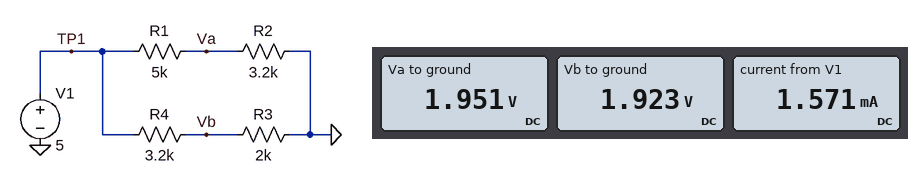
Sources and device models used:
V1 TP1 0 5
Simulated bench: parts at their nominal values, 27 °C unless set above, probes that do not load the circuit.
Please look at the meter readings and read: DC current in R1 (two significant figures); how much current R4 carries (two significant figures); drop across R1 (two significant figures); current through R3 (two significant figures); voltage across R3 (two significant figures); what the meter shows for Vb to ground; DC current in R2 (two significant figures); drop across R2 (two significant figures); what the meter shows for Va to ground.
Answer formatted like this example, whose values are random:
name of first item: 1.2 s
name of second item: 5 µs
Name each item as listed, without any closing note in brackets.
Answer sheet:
DC current in R1: 610 µA
how much current R4 carries: 960 µA
drop across R1: 3.0 V
current through R3: 960 µA
voltage across R3: 1.9 V
what the meter shows for Vb to ground: 1.923 V
DC current in R2: 610 µA
drop across R2: 2.0 V
what the meter shows for Va to ground: 1.951 V
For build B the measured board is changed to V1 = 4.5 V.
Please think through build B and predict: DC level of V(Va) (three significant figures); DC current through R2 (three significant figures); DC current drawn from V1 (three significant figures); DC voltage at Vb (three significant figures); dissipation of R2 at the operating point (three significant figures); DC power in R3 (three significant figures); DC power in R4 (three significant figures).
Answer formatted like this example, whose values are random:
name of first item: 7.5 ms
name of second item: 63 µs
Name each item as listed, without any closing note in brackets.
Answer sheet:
DC level of V(Va): 1.76 V
DC current through R2: 549 µA
DC current drawn from V1: 1.41 mA
DC voltage at Vb: 1.73 V
dissipation of R2 at the operating point: 964 µW
DC power in R3: 1.50 mW
DC power in R4: 2.40 mW
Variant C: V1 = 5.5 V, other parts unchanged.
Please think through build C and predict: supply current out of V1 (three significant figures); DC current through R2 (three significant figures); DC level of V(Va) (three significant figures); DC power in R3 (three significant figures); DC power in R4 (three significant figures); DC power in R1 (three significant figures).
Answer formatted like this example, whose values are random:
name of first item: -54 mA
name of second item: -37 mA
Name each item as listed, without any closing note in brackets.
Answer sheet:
supply current out of V1: 1.73 mA
DC current through R2: 671 µA
DC level of V(Va): 2.15 V
DC power in R3: 2.24 mW
DC power in R4: 3.58 mW
DC power in R1: 2.25 mW
